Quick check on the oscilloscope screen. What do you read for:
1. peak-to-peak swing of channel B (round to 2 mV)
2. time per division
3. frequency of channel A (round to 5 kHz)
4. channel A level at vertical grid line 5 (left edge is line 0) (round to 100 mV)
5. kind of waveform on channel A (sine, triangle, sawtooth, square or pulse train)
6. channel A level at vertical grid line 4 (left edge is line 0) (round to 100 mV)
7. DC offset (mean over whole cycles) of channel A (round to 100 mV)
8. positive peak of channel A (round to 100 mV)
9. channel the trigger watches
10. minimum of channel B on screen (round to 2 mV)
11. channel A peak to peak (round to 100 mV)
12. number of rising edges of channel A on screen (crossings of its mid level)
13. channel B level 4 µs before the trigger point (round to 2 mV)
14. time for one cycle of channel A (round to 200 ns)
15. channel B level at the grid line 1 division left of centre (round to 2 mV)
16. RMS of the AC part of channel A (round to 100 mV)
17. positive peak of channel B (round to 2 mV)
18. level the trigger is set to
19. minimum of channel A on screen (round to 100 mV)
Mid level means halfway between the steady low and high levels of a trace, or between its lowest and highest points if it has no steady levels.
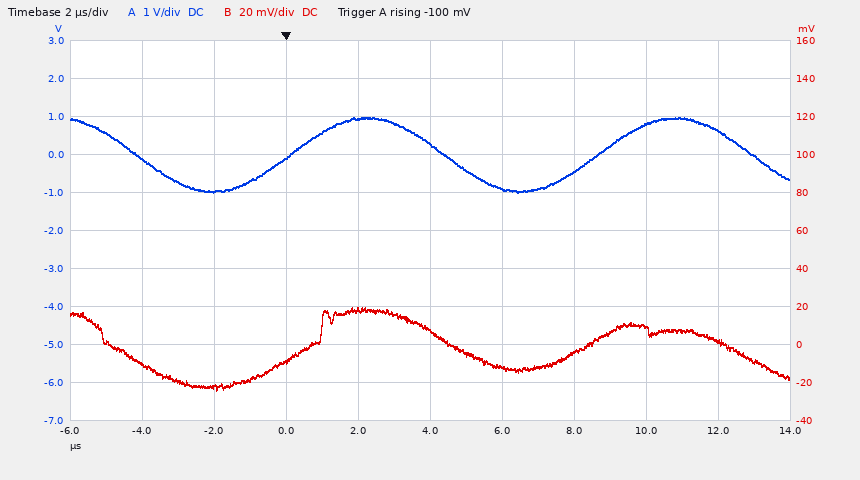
44 mV
2 µs
115 kHz
300 mV
sine
900 mV
0.0 V
1.0 V
channel A
-24 mV
2.0 V
2
-10 mV
8.6 µs
18 mV
700 mV
20 mV
-100 mV
-1.0 V
